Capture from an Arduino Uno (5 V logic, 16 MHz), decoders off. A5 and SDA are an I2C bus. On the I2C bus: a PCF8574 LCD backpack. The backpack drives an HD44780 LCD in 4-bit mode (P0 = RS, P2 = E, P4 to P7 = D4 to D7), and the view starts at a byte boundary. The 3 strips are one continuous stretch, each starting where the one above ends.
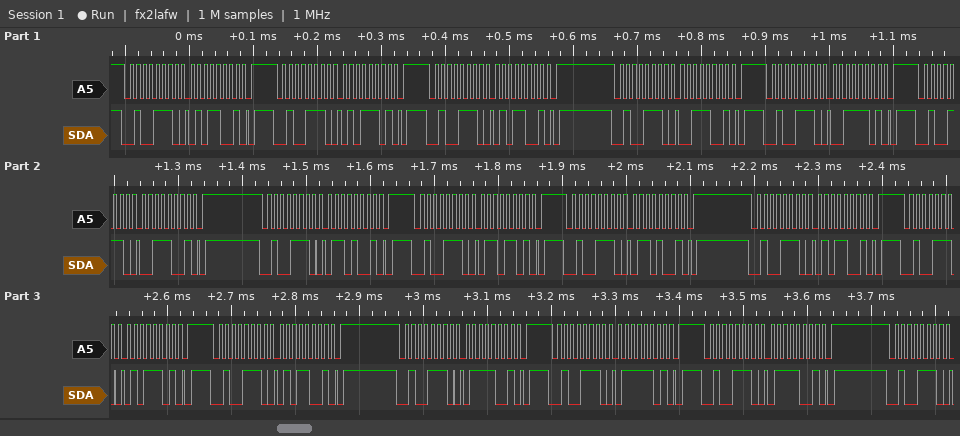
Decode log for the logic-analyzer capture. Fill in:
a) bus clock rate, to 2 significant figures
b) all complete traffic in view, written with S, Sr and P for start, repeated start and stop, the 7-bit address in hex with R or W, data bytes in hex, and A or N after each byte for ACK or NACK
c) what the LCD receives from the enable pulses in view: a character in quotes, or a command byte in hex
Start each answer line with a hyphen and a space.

- 100 kHz
- S 27W A 59 A P S 27W A 5D A P S 27W A 59 A P S 27W A 39 A P S 27W A 3D A P S 27W A 39 A P S 27W A 69 A P S 27W A 6D A P S 27W A 69 A P S 27W A 59 A P S 27W A 5D A P S 27W A 59 A P S 27W A 79 A P S 27W A 7D A P S 27W A 79 A P S 27W A
- 'S' 'e'
